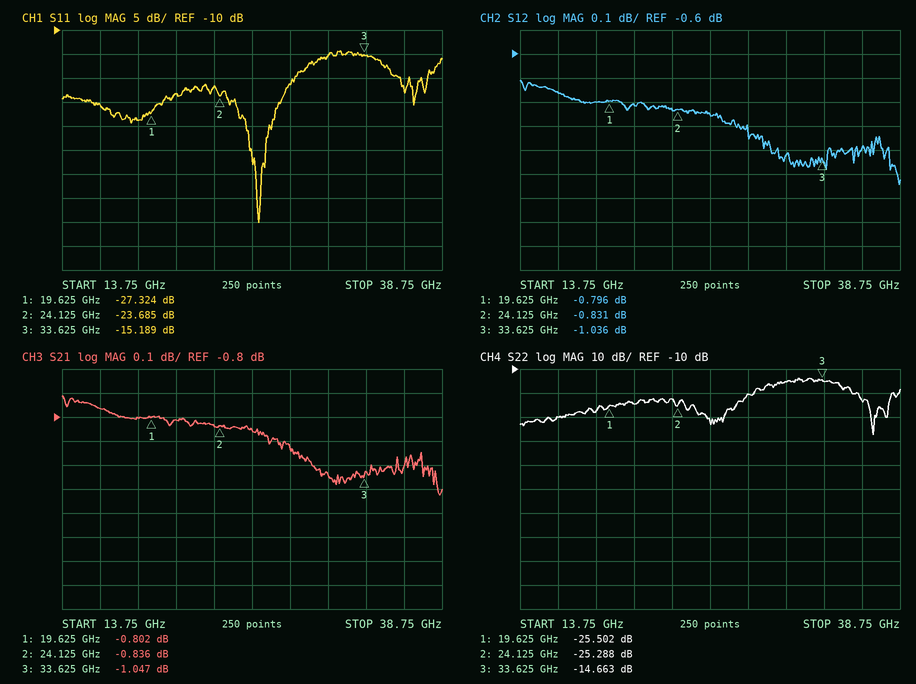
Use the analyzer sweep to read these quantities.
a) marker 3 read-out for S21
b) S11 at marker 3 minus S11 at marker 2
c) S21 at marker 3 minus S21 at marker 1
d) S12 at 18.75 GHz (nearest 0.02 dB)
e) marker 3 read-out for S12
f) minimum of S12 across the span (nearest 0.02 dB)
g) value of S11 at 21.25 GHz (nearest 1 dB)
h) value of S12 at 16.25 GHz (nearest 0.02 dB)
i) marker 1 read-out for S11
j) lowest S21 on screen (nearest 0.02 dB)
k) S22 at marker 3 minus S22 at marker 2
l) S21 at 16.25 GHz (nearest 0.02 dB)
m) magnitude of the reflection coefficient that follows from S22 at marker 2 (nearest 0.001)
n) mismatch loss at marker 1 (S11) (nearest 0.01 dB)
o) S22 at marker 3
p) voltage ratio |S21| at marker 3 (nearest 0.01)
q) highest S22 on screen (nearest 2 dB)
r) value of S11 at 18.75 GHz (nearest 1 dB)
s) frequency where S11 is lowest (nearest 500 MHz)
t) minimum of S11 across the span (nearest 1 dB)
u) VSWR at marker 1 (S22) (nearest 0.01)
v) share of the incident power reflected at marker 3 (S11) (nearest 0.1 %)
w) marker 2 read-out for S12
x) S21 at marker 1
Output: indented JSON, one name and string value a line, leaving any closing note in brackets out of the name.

{
  "marker 3 read-out for S21": "-1.047 dB",
  "S11 at marker 3 minus S11 at marker 2": "8.496 dB",
  "S21 at marker 3 minus S21 at marker 1": "-0.245 dB",
  "S12 at 18.75 GHz": "-0.80 dB",
  "marker 3 read-out for S12": "-1.036 dB",
  "minimum of S12 across the span": "-1.14 dB",
  "value of S11 at 21.25 GHz": "-23 dB",
  "value of S12 at 16.25 GHz": "-0.76 dB",
  "marker 1 read-out for S11": "-27.324 dB",
  "lowest S21 on screen": "-1.12 dB",
  "S22 at marker 3 minus S22 at marker 2": "10.625 dB",
  "S21 at 16.25 GHz": "-0.76 dB",
  "magnitude of the reflection coefficient that follows from S22 at marker 2": "0.054",
  "mismatch loss at marker 1 (S11)": "0.01 dB",
  "S22 at marker 3": "-14.663 dB",
  "voltage ratio |S21| at marker 3": "0.89",
  "highest S22 on screen": "-14 dB",
  "value of S11 at 18.75 GHz": "-29 dB",
  "frequency where S11 is lowest": "26.5 GHz",
  "minimum of S11 across the span": "-50 dB",
  "VSWR at marker 1 (S22)": "1.11",
  "share of the incident power reflected at marker 3 (S11)": "3.0 %",
  "marker 2 read-out for S12": "-0.831 dB",
  "S21 at marker 1": "-0.802 dB"
}
